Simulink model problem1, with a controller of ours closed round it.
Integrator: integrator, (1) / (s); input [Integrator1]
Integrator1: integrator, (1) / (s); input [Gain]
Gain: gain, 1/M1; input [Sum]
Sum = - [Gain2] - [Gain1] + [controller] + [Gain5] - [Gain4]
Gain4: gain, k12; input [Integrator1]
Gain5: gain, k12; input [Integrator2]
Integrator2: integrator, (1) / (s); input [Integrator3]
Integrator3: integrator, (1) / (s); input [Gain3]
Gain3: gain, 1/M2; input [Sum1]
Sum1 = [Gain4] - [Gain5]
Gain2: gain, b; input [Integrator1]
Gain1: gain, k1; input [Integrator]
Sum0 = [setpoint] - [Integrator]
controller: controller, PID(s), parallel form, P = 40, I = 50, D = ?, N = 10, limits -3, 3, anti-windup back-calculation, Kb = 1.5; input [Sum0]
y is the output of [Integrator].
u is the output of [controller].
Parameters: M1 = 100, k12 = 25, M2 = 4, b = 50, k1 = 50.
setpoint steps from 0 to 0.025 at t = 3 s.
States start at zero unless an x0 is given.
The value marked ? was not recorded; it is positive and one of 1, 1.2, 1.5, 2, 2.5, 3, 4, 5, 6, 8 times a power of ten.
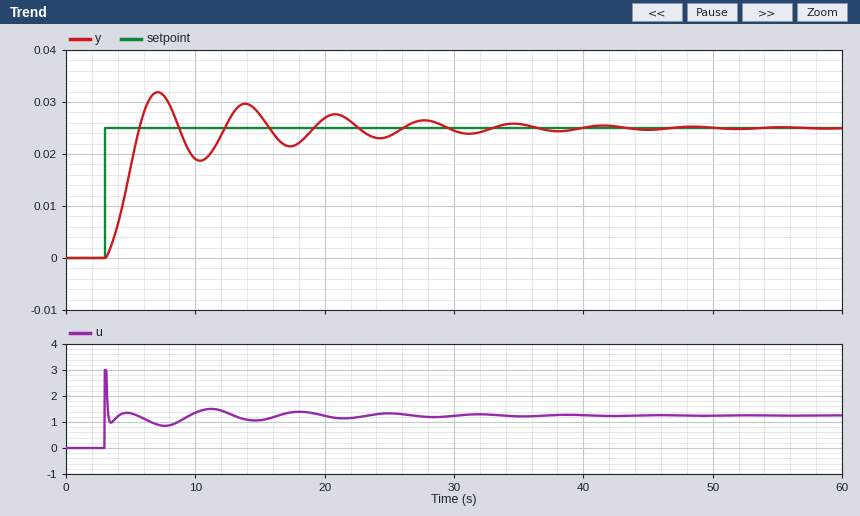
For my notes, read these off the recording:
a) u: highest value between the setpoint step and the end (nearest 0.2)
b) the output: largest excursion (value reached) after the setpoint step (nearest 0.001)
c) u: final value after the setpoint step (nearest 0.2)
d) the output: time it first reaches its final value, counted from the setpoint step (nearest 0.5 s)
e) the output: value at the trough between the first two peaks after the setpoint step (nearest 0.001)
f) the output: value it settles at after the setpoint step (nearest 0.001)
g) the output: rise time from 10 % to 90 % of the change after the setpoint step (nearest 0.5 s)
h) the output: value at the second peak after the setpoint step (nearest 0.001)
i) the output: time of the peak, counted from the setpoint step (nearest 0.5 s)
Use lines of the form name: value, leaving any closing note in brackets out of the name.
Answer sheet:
u: highest value between the setpoint step and the end: 3.0
the output: largest excursion (value reached) after the setpoint step: 0.032
u: final value after the setpoint step: 1.2
the output: time it first reaches its final value, counted from the setpoint step: 2.5 s
the output: value at the trough between the first two peaks after the setpoint step: 0.019
the output: value it settles at after the setpoint step: 0.025
the output: rise time from 10 % to 90 % of the change after the setpoint step: 2.0 s
the output: value at the second peak after the setpoint step: 0.030
the output: time of the peak, counted from the setpoint step: 4.0 s
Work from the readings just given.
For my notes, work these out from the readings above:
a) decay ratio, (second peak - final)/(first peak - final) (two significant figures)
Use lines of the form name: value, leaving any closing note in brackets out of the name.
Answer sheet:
decay ratio, (second peak - final)/(first peak - final): 0.71
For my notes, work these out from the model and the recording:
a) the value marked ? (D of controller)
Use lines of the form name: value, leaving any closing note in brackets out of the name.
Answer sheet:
the value marked ?: 30
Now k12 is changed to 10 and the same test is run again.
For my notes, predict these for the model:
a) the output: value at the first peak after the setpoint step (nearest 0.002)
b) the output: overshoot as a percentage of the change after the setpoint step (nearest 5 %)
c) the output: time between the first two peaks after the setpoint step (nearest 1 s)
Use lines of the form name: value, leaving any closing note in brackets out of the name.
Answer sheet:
the output: value at the first peak after the setpoint step: 0.032
the output: overshoot as a percentage of the change after the setpoint step: 30 %
the output: time between the first two peaks after the setpoint step: 7 s
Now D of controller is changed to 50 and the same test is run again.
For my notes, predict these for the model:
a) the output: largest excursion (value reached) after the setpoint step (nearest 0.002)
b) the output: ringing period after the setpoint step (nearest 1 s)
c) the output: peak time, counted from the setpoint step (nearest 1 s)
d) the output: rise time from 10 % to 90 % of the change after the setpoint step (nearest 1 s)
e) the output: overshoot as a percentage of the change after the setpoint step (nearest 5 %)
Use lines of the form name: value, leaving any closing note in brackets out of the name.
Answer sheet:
the output: largest excursion (value reached) after the setpoint step: 0.030
the output: ringing period after the setpoint step: 7 s
the output: peak time, counted from the setpoint step: 5 s
the output: rise time from 10 % to 90 % of the change after the setpoint step: 3 s
the output: overshoot as a percentage of the change after the setpoint step: 20 %
